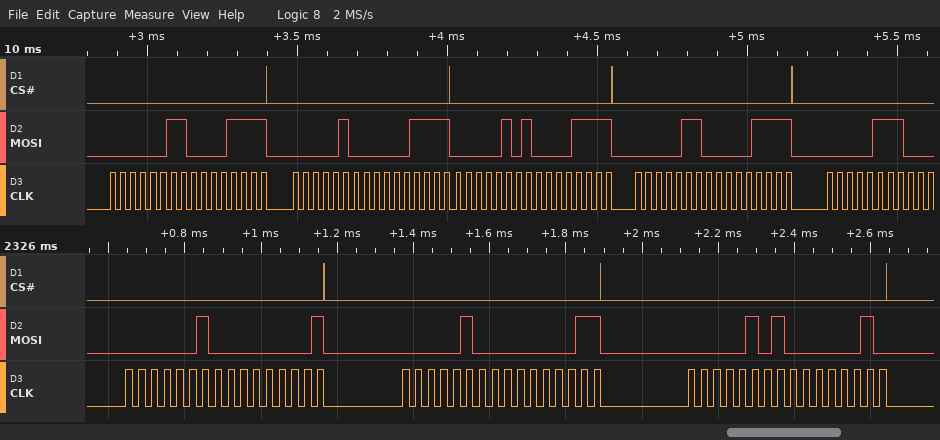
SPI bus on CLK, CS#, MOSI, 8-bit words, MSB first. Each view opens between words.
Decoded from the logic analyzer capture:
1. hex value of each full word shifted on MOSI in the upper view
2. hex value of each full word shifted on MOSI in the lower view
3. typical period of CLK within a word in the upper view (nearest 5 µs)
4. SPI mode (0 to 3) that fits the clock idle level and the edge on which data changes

03, 0F, 04, 0F, 05, 0F, 06, 0F, 07
02, 01, 04, 03, 05, 02
35 µs
0
